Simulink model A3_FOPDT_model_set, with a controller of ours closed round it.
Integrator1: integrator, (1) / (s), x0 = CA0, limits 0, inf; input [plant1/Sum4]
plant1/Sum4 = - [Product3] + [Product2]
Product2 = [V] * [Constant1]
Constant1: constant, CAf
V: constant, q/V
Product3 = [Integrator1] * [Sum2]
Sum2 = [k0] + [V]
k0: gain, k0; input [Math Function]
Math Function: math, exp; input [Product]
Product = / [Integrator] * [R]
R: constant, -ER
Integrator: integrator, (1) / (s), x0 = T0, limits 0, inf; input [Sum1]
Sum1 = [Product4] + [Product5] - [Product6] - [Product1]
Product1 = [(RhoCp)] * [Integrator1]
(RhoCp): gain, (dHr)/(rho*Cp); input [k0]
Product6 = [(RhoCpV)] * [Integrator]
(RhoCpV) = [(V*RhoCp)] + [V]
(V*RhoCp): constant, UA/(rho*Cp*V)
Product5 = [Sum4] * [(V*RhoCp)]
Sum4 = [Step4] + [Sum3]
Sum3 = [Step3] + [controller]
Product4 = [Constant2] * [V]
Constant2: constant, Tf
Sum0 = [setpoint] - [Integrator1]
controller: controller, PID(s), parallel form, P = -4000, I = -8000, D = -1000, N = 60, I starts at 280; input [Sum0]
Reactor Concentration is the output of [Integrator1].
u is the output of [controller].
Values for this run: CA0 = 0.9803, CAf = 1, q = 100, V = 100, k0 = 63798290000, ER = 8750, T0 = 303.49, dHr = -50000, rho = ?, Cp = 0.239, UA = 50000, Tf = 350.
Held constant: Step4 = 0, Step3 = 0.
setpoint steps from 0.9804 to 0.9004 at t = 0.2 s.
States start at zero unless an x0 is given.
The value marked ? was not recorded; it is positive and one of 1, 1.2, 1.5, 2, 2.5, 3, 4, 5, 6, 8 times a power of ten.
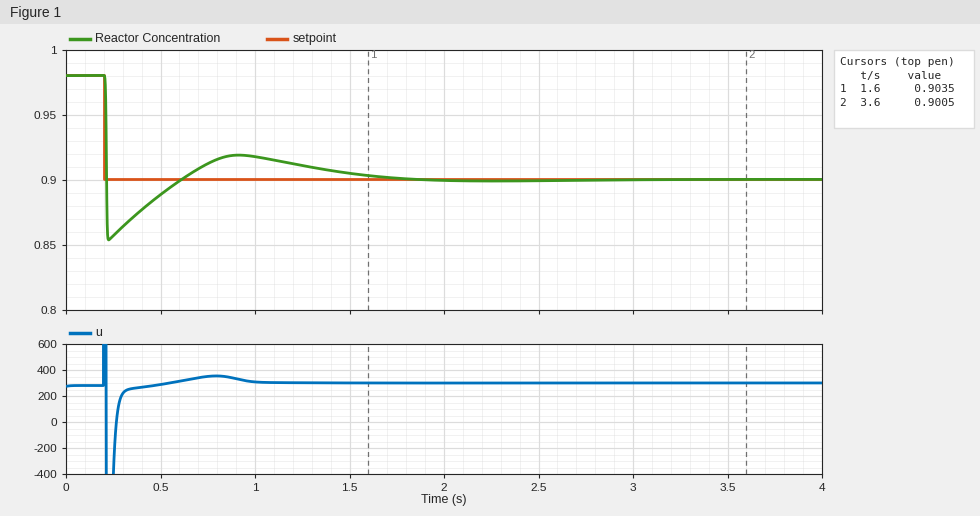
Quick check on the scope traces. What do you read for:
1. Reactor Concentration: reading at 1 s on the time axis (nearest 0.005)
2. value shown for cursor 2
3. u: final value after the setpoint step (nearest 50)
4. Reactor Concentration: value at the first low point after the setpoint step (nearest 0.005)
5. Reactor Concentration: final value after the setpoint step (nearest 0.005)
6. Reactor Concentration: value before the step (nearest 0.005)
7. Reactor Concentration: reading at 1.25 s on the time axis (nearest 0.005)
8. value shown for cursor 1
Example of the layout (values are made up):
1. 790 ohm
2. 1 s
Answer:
1. 0.920
2. 0.9005
3. 300
4. 0.855
5. 0.900
6. 0.980
7. 0.910
8. 0.9035
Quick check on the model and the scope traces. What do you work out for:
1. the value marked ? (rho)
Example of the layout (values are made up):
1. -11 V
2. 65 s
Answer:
1. 1000
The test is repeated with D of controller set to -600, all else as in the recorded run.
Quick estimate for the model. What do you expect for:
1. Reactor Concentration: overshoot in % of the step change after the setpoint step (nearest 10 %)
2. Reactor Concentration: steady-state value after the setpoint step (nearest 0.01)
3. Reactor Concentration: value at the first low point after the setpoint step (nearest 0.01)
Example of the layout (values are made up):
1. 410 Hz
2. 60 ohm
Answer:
1. 30 %
2. 0.90
3. 0.88
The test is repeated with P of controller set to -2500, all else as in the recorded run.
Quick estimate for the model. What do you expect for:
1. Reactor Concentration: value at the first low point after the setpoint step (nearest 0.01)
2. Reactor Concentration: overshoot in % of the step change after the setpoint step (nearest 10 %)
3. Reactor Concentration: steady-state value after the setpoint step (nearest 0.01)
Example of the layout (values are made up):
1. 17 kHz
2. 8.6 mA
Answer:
1. 0.86
2. 50 %
3. 0.90
